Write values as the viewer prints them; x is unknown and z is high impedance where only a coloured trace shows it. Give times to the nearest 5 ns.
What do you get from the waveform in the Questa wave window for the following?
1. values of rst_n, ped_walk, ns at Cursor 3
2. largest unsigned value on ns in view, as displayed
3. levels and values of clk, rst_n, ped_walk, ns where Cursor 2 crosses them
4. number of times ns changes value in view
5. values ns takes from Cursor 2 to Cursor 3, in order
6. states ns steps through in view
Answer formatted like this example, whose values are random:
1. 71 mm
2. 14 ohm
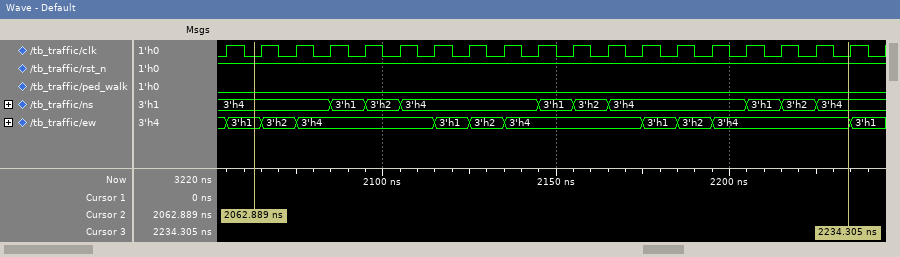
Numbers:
1. rst_n=1, ped_walk=0, ns=3'h4
2. 3'h4
3. clk=0, rst_n=1, ped_walk=0, ns=3'h4
4. 9
5. 3'h4, 3'h1, 3'h2, 3'h4, 3'h1, 3'h2, 3'h4, 3'h1, 3'h2, 3'h4
6. 3'h4, 3'h1, 3'h2, 3'h4, 3'h1, 3'h2, 3'h4, 3'h1, 3'h2, 3'h4
